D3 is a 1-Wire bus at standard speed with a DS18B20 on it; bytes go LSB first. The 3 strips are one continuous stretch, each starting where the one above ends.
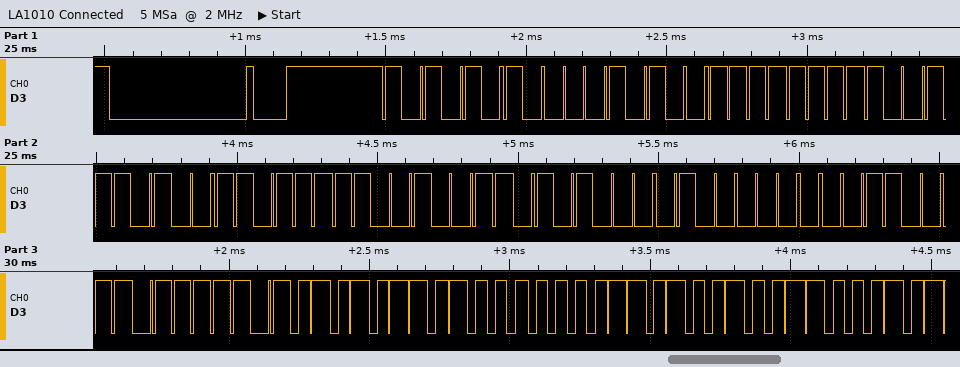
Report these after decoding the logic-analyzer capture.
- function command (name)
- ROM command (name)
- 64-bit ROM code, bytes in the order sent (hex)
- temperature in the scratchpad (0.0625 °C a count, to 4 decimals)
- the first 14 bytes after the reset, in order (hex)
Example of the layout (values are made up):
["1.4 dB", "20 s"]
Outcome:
["Read Scratchpad", "Match ROM", "28 FF B9 EC 93 15 02 CC", "22.6250 °C", "55 28 FF B9 EC 93 15 02 CC BE 6A 01 4B 46"]
